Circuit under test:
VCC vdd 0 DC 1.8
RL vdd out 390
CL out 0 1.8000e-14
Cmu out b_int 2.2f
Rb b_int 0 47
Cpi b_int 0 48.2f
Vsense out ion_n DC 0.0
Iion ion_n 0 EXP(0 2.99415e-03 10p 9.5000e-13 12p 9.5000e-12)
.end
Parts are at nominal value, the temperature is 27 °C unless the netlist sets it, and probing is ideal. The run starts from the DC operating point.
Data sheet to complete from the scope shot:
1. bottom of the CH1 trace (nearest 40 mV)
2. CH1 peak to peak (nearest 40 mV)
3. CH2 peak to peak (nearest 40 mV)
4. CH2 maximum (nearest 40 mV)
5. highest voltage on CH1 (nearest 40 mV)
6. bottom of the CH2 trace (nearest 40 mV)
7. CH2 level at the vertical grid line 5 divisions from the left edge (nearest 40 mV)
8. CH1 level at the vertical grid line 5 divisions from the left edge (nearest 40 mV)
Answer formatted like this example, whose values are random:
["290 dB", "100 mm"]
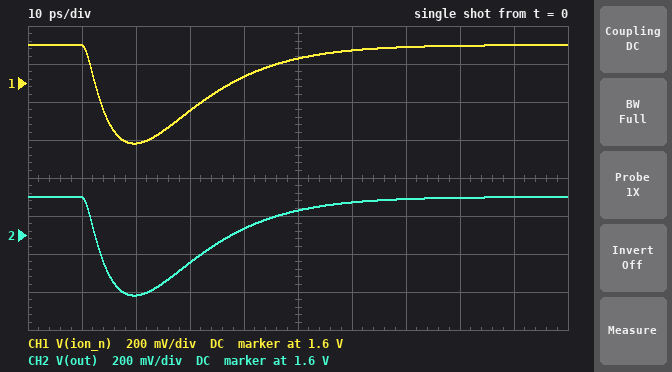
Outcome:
["1.28 V", "520 mV", "520 mV", "1.80 V", "1.80 V", "1.28 V", "1.72 V", "1.72 V"]
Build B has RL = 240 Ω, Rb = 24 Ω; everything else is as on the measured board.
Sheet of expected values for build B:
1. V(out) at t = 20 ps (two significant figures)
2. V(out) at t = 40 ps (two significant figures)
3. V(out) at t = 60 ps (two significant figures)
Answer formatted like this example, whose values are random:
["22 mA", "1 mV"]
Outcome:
["1.4 V", "1.7 V", "1.8 V"]
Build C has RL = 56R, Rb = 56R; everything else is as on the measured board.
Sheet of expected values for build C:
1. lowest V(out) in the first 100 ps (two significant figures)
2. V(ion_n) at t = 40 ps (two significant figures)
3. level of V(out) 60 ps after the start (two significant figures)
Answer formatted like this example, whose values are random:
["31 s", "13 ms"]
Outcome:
["1.7 V", "1.8 V", "1.8 V"]
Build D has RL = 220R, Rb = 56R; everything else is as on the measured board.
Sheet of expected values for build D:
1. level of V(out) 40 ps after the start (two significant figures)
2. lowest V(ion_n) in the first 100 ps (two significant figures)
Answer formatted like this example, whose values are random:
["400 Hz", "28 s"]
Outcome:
["1.7 V", "1.4 V"]
